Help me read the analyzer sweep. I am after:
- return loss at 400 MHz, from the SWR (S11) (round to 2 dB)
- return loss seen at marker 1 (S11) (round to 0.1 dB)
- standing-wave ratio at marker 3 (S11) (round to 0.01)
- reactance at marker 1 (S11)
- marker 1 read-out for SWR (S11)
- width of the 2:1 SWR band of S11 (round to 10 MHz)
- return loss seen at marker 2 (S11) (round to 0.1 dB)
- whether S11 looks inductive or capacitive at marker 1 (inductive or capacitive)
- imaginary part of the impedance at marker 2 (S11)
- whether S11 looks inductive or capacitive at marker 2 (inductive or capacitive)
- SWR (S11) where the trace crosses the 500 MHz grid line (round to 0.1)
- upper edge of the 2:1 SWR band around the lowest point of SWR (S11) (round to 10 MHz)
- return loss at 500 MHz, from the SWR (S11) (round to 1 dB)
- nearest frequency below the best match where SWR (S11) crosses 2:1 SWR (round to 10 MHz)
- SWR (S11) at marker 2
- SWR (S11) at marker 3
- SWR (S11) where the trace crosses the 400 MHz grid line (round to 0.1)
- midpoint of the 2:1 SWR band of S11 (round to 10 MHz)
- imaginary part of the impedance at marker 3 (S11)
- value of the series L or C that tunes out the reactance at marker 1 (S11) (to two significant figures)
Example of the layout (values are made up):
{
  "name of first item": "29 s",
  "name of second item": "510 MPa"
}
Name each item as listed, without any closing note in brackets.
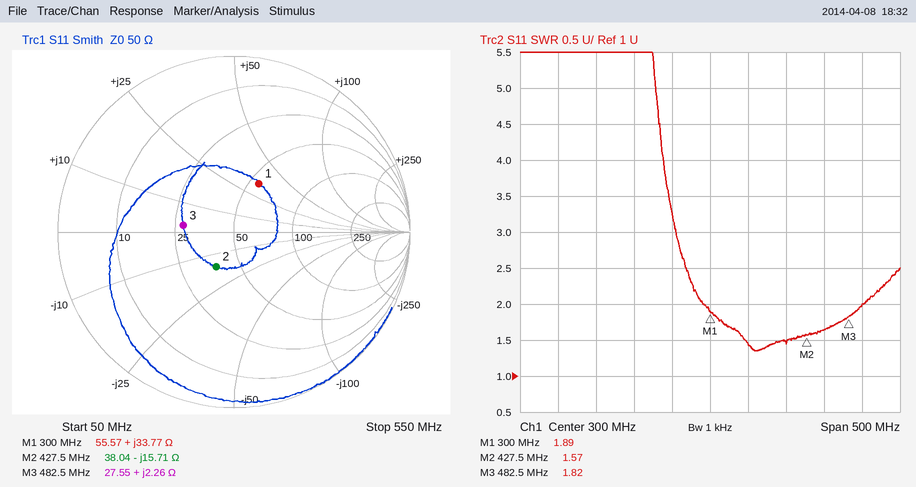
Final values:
{
  "return loss at 400 MHz, from the SWR (S11)": "14 dB",
  "return loss seen at marker 1 (S11)": "10.2 dB",
  "standing-wave ratio at marker 3 (S11)": "1.82",
  "reactance at marker 1": "+33.77 Ω",
  "marker 1 read-out for SWR": "1.89",
  "width of the 2:1 SWR band of S11": "210 MHz",
  "return loss seen at marker 2 (S11)": "13.1 dB",
  "whether S11 looks inductive or capacitive at marker 1": "inductive",
  "imaginary part of the impedance at marker 2": "-15.71 Ω",
  "whether S11 looks inductive or capacitive at marker 2": "capacitive",
  "SWR (S11) where the trace crosses the 500 MHz grid line": "2.0",
  "upper edge of the 2:1 SWR band around the lowest point of SWR (S11)": "500 MHz",
  "return loss at 500 MHz, from the SWR (S11)": "10 dB",
  "nearest frequency below the best match where SWR (S11) crosses 2:1 SWR": "290 MHz",
  "SWR (S11) at marker 2": "1.57",
  "SWR (S11) at marker 3": "1.82",
  "SWR (S11) where the trace crosses the 400 MHz grid line": "1.5",
  "midpoint of the 2:1 SWR band of S11": "400 MHz",
  "imaginary part of the impedance at marker 3": "+2.26 Ω",
  "value of the series L or C that tunes out the reactance at marker 1 (S11)": "16 pF"
}
